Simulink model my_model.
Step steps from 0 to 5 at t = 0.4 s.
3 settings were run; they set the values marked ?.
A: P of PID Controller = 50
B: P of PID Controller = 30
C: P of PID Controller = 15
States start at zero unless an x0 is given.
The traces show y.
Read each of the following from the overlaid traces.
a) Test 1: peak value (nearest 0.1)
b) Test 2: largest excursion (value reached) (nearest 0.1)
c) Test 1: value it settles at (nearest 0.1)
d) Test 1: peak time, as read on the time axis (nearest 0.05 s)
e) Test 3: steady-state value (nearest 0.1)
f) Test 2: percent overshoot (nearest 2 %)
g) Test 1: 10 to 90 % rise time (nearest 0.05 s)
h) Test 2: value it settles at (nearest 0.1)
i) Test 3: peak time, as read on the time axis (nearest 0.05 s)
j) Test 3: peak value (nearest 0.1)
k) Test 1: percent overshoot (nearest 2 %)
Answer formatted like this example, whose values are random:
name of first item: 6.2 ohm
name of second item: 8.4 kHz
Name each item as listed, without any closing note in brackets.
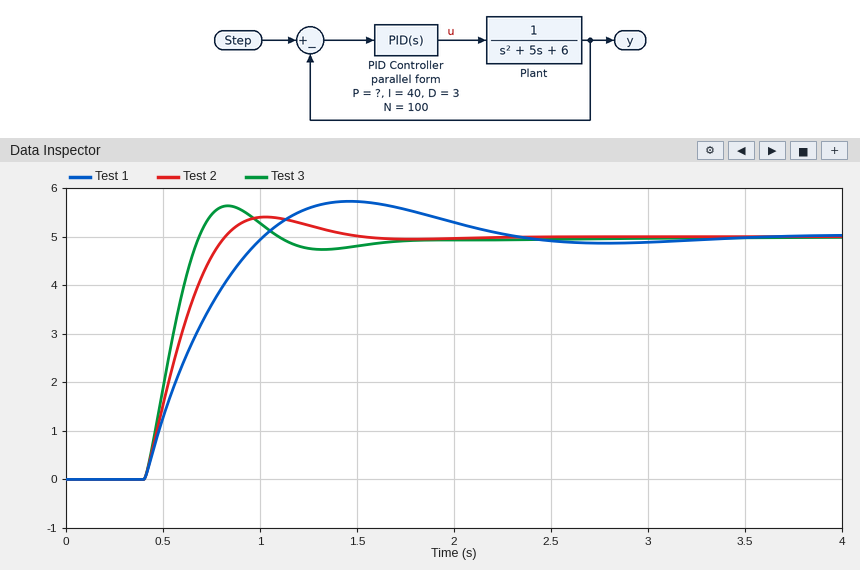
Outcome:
Test 1: peak value: 5.7
Test 2: largest excursion (value reached): 5.4
Test 1: value it settles at: 5.0
Test 1: peak time, as read on the time axis: 1.45 s
Test 3: steady-state value: 5.0
Test 2: percent overshoot: 8 %
Test 1: 10 to 90 % rise time: 0.45 s
Test 2: value it settles at: 5.0
Test 3: peak time, as read on the time axis: 0.85 s
Test 3: peak value: 5.6
Test 1: percent overshoot: 14 %
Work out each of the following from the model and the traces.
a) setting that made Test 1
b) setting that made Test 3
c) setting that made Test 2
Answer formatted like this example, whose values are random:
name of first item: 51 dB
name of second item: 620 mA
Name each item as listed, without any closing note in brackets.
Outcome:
setting that made Test 1: C
setting that made Test 3: A
setting that made Test 2: B
